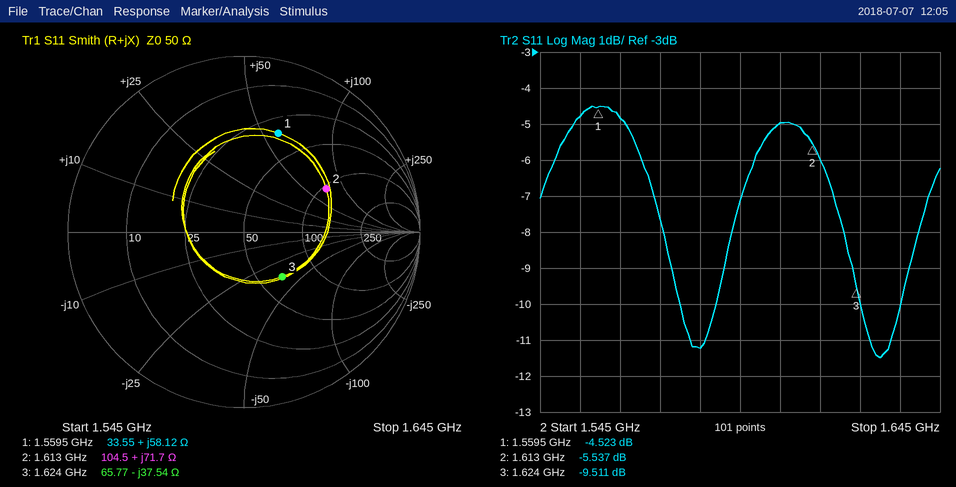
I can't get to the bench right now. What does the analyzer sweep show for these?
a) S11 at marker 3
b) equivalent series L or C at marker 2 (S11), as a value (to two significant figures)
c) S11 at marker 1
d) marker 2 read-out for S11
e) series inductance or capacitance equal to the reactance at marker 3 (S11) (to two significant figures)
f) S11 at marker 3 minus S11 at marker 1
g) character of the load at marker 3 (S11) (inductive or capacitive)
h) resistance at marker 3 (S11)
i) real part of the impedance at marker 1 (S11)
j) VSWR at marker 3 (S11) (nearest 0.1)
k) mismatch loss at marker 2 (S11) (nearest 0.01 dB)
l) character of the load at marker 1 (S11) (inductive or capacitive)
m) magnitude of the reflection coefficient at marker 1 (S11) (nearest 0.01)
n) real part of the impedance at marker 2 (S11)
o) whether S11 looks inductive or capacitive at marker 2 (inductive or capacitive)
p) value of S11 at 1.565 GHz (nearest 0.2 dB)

-9.511 dB
7.1 nH
-4.523 dB
-5.537 dB
2.6 pF
-4.988 dB
capacitive
65.77 Ω
33.55 Ω
2.0
1.42 dB
inductive
0.59
104.5 Ω
inductive
-4.8 dB
